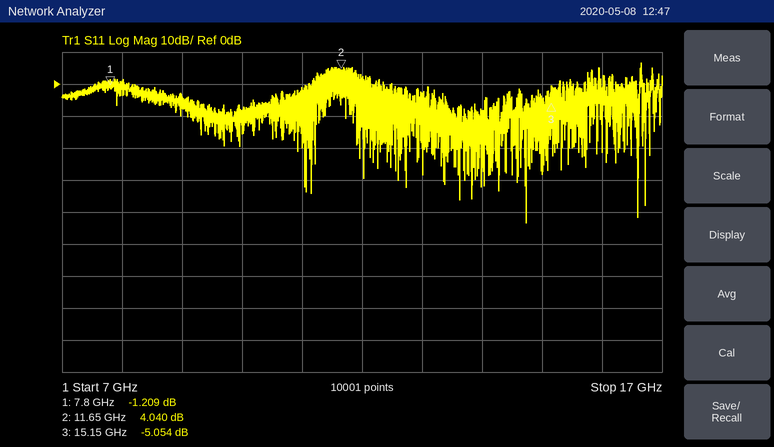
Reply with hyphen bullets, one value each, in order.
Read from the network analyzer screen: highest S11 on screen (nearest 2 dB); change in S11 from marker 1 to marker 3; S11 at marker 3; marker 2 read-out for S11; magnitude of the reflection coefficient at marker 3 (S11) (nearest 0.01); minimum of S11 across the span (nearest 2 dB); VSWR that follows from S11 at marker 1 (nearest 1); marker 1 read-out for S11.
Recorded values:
- 6 dB
- -3.845 dB
- -5.054 dB
- 4.040 dB
- 0.56
- -44 dB
- 14
- -1.209 dB
